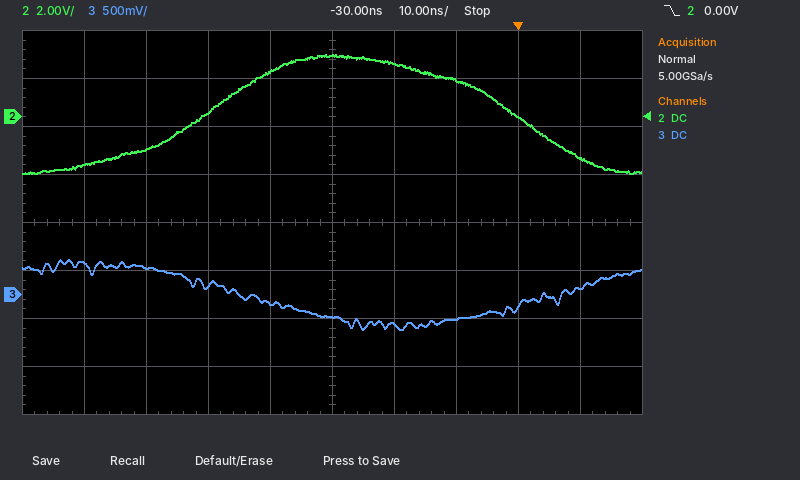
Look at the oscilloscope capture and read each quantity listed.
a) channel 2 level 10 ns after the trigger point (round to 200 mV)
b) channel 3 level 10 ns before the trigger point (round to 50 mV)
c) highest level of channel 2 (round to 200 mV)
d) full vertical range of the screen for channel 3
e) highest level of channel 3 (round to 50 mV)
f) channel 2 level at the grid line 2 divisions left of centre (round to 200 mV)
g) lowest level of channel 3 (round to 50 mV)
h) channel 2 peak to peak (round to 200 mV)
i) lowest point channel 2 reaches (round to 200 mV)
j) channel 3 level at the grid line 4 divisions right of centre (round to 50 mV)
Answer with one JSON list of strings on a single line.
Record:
["-1.8 V", "-250 mV", "2.6 V", "4 V", "350 mV", "200 mV", "-350 mV", "5.0 V", "-2.4 V", "50 mV"]
